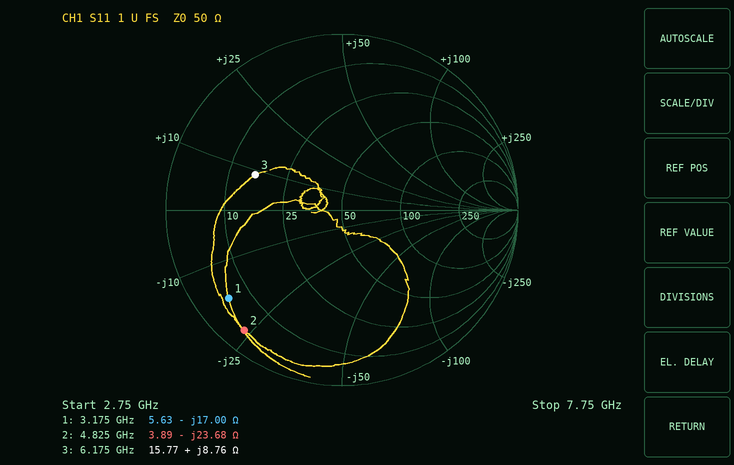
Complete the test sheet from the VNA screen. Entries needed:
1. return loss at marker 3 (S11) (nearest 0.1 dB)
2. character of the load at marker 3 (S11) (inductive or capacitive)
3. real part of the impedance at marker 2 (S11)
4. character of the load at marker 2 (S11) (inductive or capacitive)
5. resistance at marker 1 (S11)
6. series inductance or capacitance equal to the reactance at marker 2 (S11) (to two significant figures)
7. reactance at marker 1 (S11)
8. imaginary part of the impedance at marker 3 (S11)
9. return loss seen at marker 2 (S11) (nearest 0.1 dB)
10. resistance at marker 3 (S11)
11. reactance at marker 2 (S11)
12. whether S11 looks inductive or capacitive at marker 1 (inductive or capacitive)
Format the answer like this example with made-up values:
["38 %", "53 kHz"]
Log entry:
["5.5 dB", "inductive", "3.89 Ω", "capacitive", "5.63 Ω", "1.4 pF", "-17.00 Ω", "+8.76 Ω", "1.1 dB", "15.77 Ω", "-23.68 Ω", "capacitive"]
